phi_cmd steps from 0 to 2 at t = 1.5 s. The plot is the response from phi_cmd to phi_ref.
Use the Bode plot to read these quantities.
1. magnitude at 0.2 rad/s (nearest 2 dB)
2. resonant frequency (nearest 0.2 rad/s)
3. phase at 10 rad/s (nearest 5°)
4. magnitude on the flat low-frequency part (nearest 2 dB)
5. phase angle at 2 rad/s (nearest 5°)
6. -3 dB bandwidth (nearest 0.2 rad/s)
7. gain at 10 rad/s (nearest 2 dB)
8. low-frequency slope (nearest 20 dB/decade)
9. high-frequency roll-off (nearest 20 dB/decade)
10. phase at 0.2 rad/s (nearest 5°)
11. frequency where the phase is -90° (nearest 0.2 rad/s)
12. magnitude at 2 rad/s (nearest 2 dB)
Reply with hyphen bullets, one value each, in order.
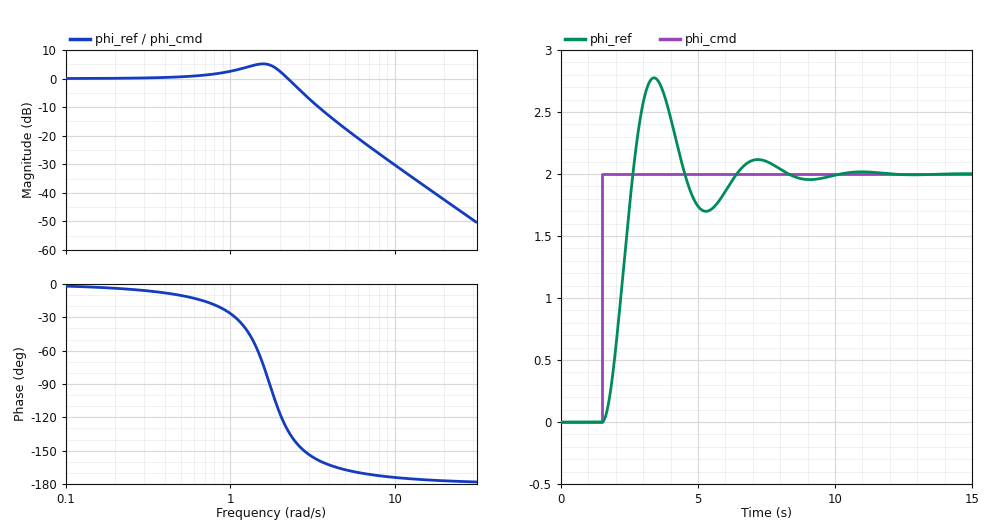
- 0 dB
- 1.6 rad/s
- -175°
- 0 dB
- -115°
- 2.6 rad/s
- -30 dB
- 0 dB/decade
- -40 dB/decade
- -5°
- 1.8 rad/s
- 2 dB
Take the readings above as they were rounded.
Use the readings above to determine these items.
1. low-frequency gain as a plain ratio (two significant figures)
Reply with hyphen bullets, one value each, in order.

- 1.0
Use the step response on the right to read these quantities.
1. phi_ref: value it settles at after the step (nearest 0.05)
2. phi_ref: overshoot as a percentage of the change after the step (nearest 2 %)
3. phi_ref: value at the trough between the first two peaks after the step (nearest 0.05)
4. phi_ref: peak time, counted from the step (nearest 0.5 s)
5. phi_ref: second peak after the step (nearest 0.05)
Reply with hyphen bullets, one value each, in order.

- 2.00
- 38 %
- 1.70
- 2.0 s
- 2.10
